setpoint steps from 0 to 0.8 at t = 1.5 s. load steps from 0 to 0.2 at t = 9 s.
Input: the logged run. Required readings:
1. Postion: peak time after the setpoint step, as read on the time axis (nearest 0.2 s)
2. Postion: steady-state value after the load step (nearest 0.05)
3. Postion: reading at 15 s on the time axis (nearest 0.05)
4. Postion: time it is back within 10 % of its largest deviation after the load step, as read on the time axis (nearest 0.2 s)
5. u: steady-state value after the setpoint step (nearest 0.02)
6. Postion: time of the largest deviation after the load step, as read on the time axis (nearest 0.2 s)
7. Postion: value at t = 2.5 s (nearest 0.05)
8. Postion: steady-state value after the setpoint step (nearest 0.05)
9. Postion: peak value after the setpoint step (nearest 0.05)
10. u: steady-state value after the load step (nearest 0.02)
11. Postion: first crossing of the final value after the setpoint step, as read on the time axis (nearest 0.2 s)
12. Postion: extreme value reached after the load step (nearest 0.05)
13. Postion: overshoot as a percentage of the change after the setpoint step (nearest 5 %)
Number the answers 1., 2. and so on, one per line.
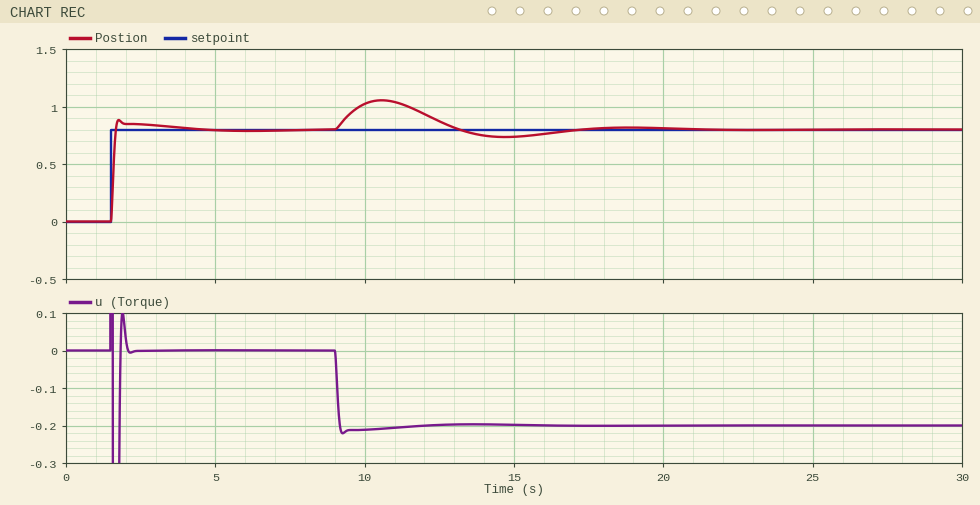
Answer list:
1. 1.8 s
2. 0.80
3. 0.75
4. 16.4 s
5. 0.00
6. 10.6 s
7. 0.85
8. 0.80
9. 0.90
10. -0.20
11. 1.6 s
12. 1.05
13. 10 %
